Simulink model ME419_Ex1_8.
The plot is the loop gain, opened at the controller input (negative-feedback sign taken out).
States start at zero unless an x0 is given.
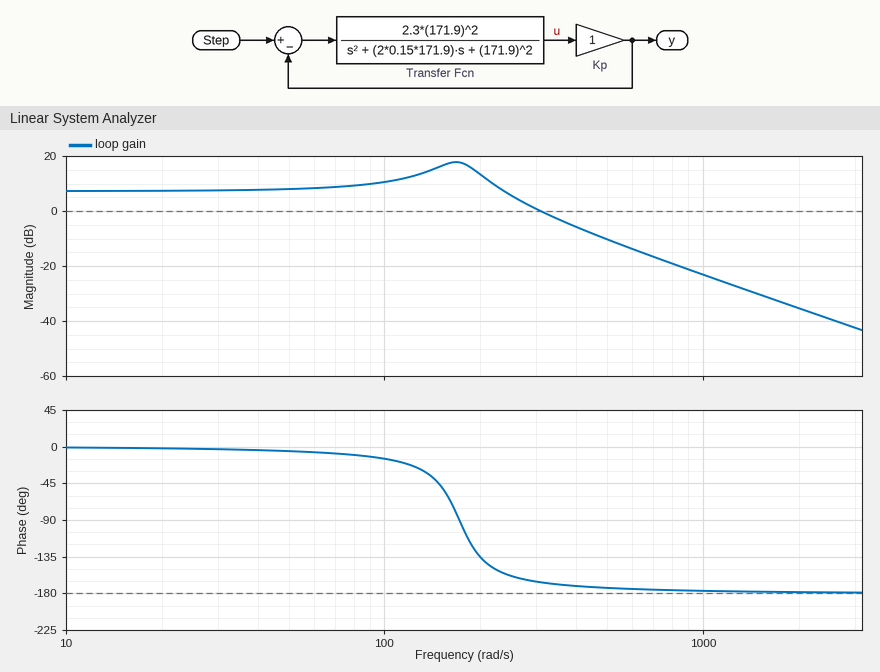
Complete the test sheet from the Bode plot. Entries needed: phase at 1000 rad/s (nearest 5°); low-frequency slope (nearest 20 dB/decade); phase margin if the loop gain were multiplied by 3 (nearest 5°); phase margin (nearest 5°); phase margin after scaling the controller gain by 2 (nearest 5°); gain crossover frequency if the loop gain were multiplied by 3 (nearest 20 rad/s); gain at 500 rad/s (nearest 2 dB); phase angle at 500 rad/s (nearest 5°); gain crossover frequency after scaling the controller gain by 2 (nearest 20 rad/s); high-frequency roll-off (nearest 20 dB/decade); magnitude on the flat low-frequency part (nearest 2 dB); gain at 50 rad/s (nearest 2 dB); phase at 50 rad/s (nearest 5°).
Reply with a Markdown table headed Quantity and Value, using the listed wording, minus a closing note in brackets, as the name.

| Quantity | Value |
|---|---|
| phase at 1000 rad/s | -175° |
| low-frequency slope | 0 dB/decade |
| phase margin if the loop gain were multiplied by 3 | 5° |
| phase margin | 15° |
| phase margin after scaling the controller gain by 2 | 10° |
| gain crossover frequency if the loop gain were multiplied by 3 | 480 rad/s |
| gain at 500 rad/s | -10 dB |
| phase angle at 500 rad/s | -175° |
| gain crossover frequency after scaling the controller gain by 2 | 400 rad/s |
| high-frequency roll-off | -40 dB/decade |
| magnitude on the flat low-frequency part | 8 dB |
| gain at 50 rad/s | 8 dB |
| phase at 50 rad/s | -5° |
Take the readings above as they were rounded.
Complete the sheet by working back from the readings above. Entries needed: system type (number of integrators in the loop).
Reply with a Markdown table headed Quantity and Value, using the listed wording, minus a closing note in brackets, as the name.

| Quantity | Value |
|---|---|
| system type | 0 |
